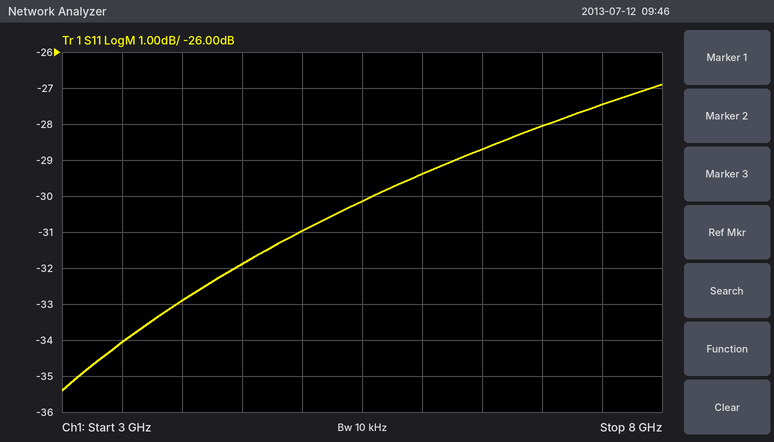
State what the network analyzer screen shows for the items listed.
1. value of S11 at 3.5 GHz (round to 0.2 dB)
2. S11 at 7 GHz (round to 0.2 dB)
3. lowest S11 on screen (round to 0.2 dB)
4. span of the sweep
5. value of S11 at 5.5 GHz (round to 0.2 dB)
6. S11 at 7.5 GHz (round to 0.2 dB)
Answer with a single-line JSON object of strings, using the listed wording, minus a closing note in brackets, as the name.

{"value of S11 at 3.5 GHz": "-34.0 dB", "S11 at 7 GHz": "-28.0 dB", "lowest S11 on screen": "-35.4 dB", "span of the sweep": "5 GHz", "value of S11 at 5.5 GHz": "-30.2 dB", "S11 at 7.5 GHz": "-27.4 dB"}
